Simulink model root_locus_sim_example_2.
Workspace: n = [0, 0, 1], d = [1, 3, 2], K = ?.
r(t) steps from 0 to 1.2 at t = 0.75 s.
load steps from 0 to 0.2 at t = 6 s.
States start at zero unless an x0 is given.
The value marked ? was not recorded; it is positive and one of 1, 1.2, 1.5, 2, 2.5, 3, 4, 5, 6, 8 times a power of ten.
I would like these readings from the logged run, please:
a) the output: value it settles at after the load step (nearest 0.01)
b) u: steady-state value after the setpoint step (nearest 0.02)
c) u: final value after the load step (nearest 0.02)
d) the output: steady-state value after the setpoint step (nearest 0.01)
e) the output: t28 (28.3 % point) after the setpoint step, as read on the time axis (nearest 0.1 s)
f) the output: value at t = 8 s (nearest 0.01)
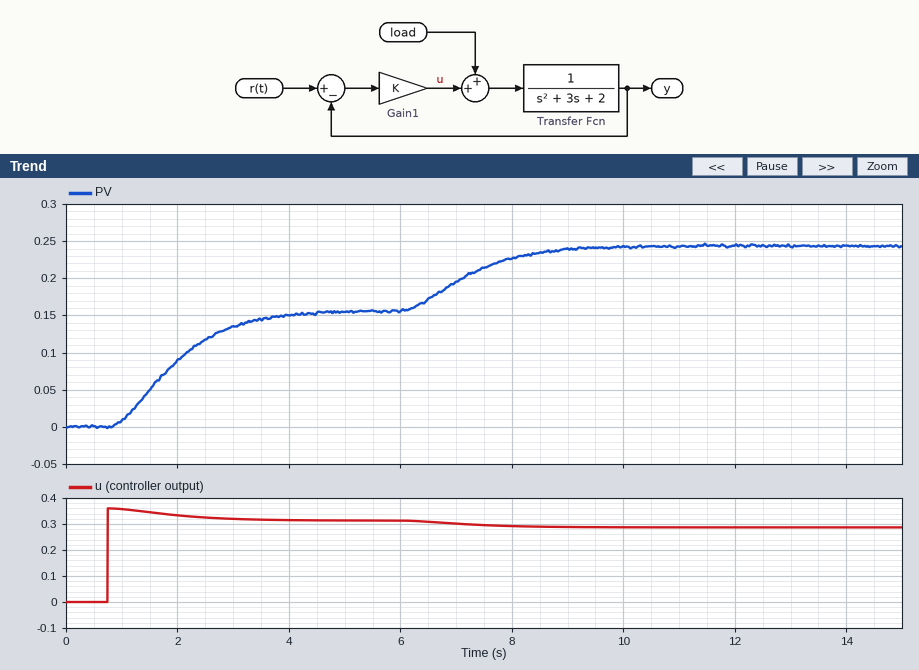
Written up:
0.24
0.32
0.28
0.16
1.4 s
0.23
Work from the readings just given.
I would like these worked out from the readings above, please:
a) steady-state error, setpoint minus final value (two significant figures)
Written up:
1.0
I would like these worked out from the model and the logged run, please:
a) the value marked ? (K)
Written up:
0.3
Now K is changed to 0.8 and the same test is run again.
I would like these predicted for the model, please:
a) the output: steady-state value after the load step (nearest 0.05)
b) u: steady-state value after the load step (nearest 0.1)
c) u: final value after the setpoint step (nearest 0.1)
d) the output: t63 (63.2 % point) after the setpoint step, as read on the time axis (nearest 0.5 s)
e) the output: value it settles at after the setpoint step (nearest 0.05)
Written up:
0.40
0.6
0.7
2.0 s
0.35
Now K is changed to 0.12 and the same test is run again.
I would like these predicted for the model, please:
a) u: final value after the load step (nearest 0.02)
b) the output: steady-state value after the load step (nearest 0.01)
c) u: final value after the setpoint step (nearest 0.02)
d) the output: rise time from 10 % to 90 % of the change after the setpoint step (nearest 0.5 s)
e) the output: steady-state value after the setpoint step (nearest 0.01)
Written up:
0.12
0.16
0.14
2.5 s
0.07
